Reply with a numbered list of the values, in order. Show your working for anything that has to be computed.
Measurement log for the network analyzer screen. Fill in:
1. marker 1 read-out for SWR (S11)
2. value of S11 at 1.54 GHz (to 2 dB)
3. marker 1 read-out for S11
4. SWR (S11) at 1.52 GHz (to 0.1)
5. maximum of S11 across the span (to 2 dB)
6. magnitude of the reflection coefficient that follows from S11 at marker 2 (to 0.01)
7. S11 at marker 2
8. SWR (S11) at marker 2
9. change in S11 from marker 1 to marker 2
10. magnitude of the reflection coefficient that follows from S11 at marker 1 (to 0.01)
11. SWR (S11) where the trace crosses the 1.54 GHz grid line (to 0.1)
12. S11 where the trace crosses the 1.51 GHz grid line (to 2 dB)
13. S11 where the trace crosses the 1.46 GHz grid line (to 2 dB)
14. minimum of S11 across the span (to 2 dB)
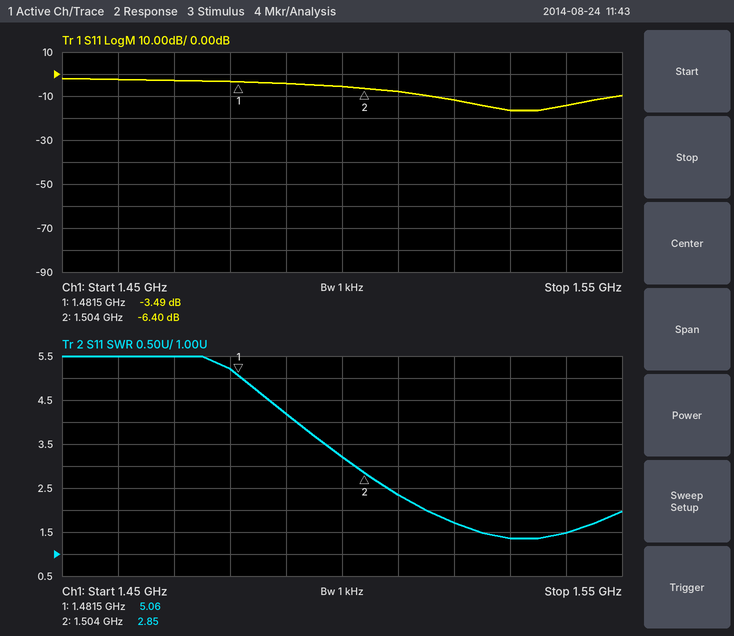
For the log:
1. 5.06
2. -14 dB
3. -3.49 dB
4. 1.7
5. -2 dB
6. 10^(-6.4/20) ≈ 0.48
7. -6.40 dB
8. 2.85
9. -6.4 − (-3.49) = -2.91 dB
10. 10^(-3.49/20) ≈ 0.67
11. 1.5
12. -8 dB
13. -2 dB
14. -16 dB
